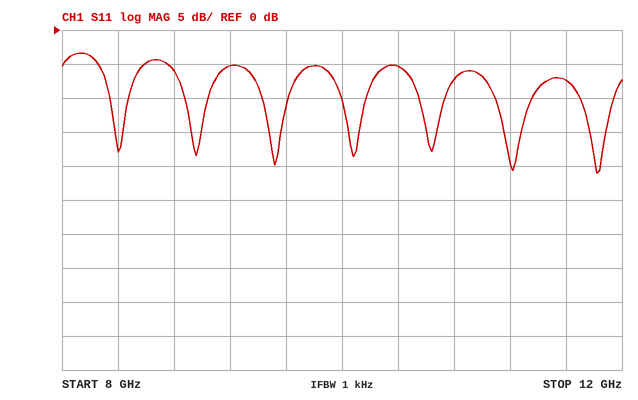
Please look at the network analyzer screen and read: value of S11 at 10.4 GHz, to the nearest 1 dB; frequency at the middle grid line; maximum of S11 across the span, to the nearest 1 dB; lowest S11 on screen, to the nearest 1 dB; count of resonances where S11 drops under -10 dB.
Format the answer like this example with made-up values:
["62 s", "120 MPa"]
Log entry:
["-5 dB", "10 GHz", "-3 dB", "-21 dB", "7"]
